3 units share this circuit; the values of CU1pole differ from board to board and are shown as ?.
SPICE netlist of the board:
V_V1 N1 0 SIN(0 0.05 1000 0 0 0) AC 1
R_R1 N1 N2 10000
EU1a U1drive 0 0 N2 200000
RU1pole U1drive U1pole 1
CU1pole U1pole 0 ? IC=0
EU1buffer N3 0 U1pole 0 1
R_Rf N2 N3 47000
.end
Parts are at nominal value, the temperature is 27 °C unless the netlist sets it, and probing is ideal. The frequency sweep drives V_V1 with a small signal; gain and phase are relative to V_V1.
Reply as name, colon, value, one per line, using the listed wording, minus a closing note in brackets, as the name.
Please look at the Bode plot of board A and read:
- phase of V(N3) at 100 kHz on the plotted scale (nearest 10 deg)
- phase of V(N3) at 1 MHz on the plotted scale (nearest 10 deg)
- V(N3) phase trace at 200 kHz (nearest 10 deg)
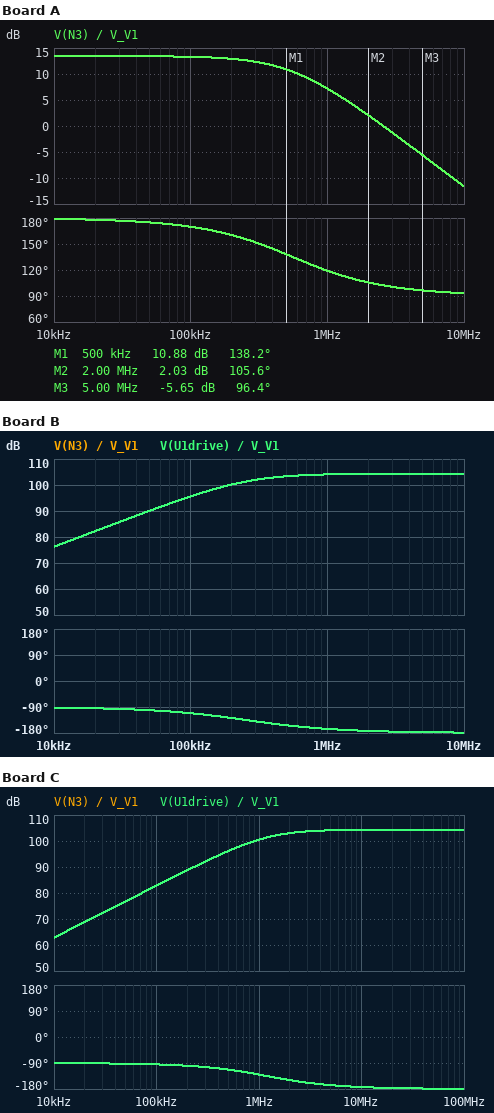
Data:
phase of V(N3) at 100 kHz on the plotted scale: 170 deg
phase of V(N3) at 1 MHz on the plotted scale: 120 deg
V(N3) phase trace at 200 kHz: 160 deg
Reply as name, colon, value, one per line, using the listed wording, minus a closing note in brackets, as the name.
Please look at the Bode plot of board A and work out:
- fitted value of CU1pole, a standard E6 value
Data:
fitted value of CU1pole, a standard E6 value: 10 mF
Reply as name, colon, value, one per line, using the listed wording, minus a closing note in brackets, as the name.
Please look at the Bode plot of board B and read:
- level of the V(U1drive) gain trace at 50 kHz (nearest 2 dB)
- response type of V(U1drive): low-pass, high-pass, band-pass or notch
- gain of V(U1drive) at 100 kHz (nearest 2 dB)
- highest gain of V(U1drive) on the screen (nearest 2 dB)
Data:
level of the V(U1drive) gain trace at 50 kHz: 90 dB
response type of V(U1drive): low-pass, high-pass, band-pass or notch: high-pass
gain of V(U1drive) at 100 kHz: 96 dB
highest gain of V(U1drive) on the screen: 104 dB
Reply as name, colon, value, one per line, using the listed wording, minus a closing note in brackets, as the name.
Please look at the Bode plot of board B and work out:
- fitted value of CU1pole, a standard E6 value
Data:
fitted value of CU1pole, a standard E6 value: 22 mF
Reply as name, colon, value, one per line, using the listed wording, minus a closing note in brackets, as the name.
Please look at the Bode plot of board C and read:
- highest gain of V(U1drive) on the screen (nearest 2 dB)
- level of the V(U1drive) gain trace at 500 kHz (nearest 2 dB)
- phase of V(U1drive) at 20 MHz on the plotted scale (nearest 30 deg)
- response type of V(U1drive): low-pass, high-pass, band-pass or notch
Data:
highest gain of V(U1drive) on the screen: 104 dB
level of the V(U1drive) gain trace at 500 kHz: 96 dB
phase of V(U1drive) at 20 MHz on the plotted scale: -180 deg
response type of V(U1drive): low-pass, high-pass, band-pass or notch: high-pass
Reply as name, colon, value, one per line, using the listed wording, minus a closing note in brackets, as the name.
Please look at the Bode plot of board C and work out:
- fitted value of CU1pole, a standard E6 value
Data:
fitted value of CU1pole, a standard E6 value: 4.7 mF
